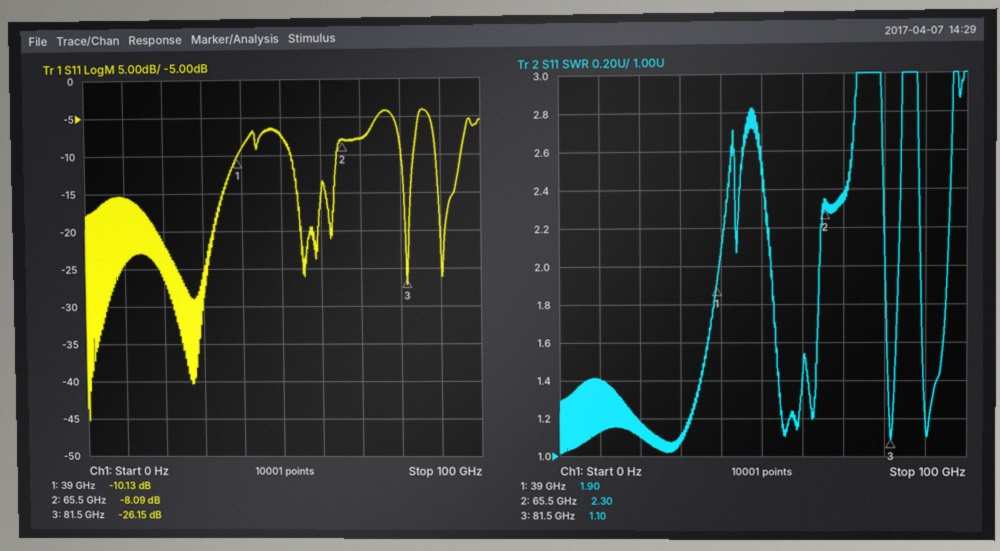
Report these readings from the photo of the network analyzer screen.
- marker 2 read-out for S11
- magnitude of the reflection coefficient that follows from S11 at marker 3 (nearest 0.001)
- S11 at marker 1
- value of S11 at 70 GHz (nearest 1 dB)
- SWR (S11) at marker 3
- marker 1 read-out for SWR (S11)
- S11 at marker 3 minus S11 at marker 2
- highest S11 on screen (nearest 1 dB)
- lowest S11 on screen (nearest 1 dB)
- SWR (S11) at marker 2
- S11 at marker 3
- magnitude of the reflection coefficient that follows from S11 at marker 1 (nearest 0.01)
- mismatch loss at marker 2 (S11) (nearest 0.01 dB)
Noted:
-8.09 dB
0.049
-10.13 dB
-8 dB
1.10
1.90
-18.06 dB
-4 dB
-45 dB
2.30
-26.15 dB
0.31
0.73 dB
